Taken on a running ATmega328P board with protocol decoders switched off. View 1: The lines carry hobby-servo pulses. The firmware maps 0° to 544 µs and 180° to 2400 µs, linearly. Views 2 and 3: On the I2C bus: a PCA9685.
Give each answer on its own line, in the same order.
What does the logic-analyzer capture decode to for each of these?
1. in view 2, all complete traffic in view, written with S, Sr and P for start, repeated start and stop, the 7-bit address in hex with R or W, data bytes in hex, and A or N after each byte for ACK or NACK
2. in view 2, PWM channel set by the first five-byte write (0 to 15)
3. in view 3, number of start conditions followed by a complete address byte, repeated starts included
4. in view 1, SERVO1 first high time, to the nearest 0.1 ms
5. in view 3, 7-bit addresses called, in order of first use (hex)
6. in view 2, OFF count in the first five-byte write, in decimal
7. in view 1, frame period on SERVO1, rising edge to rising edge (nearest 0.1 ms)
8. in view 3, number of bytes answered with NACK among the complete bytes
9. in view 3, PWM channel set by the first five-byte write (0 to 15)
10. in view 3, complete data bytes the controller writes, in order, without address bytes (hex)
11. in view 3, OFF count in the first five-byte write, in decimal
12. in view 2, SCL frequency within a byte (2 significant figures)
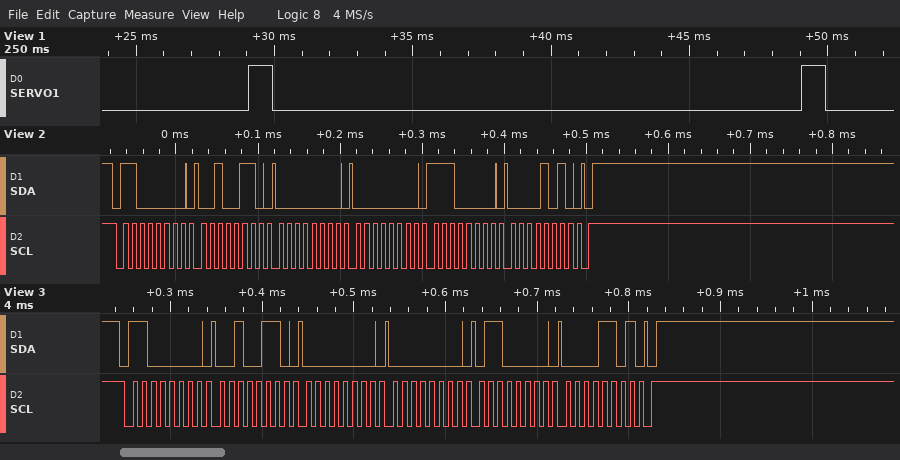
S 60W A 26 A 00 A 00 A E0 A 0A A P
8
1
0.9 ms
0x60
2784
20.0 ms
0
8
26 00 00 60 0D
3424
100 kHz
